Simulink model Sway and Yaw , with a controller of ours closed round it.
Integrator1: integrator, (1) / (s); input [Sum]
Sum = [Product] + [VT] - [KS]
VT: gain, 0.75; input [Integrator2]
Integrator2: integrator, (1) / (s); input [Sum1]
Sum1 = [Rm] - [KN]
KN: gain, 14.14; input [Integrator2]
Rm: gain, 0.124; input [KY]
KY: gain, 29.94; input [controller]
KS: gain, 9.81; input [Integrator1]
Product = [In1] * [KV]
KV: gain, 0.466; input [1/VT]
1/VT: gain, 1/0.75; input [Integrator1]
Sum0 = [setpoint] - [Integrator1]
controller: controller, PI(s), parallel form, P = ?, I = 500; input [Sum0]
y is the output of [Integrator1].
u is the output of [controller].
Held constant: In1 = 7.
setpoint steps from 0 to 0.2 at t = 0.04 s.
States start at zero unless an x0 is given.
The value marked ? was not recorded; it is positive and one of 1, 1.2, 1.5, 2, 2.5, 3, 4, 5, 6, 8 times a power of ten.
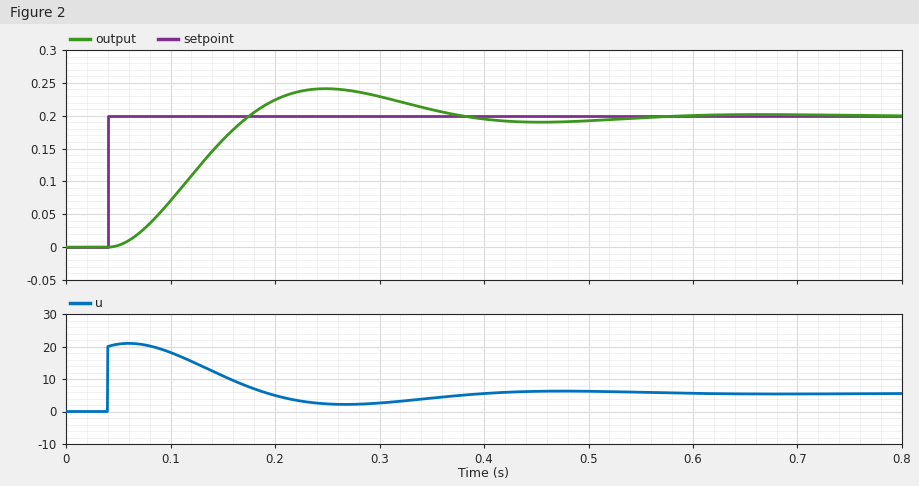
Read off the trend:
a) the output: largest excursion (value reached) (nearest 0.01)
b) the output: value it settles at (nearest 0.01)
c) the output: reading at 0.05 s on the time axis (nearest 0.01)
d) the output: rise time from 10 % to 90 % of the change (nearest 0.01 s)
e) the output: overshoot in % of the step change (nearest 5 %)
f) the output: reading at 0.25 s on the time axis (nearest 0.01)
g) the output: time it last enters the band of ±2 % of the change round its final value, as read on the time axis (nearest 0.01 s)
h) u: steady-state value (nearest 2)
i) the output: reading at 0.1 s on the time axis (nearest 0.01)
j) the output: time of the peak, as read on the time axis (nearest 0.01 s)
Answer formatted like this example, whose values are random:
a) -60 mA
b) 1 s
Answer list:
a) 0.24
b) 0.20
c) 0.00
d) 0.09 s
e) 20 %
f) 0.24
g) 0.54 s
h) 6
i) 0.07
j) 0.25 s
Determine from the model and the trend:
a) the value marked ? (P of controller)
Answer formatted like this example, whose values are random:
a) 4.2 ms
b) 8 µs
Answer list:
a) 100
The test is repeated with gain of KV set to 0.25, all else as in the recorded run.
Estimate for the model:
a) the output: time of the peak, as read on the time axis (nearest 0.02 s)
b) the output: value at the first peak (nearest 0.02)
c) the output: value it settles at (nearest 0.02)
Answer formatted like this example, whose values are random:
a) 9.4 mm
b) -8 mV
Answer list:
a) 0.26 s
b) 0.22
c) 0.20
